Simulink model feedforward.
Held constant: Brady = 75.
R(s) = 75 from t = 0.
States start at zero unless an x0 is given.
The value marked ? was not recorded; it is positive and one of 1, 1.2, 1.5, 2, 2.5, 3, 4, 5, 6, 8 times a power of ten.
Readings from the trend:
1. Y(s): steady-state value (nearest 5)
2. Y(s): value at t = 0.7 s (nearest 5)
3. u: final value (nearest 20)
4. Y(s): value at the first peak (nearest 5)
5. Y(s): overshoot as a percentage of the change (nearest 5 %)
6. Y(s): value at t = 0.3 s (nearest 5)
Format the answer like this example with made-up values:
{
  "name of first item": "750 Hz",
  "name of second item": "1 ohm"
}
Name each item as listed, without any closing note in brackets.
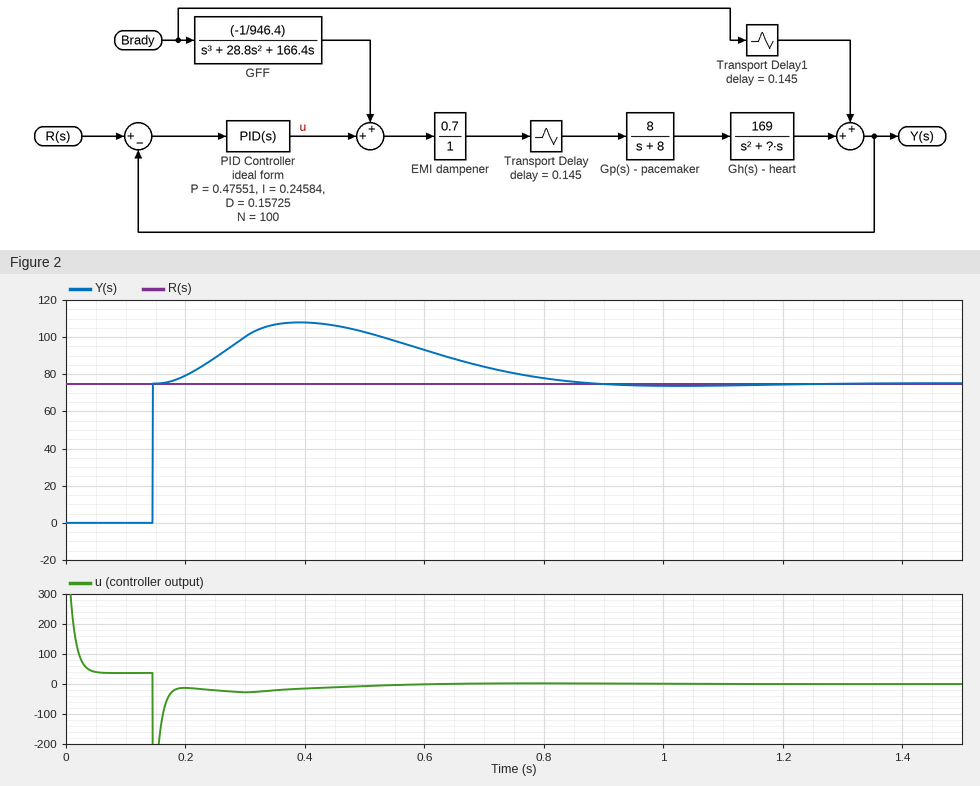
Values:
{
  "Y(s): steady-state value": "75",
  "Y(s): value at t = 0.7 s": "85",
  "u: final value": "0",
  "Y(s): value at the first peak": "110",
  "Y(s): overshoot as a percentage of the change": "45 %",
  "Y(s): value at t = 0.3 s": "100"
}
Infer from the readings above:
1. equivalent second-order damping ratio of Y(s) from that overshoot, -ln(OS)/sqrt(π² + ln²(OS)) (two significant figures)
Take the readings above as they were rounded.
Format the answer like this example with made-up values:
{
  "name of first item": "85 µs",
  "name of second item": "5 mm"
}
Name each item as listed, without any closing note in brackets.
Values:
{
  "equivalent second-order damping ratio of Y(s) from that overshoot, -ln(OS)/sqrt(π² + ln²(OS))": "0.25"
}
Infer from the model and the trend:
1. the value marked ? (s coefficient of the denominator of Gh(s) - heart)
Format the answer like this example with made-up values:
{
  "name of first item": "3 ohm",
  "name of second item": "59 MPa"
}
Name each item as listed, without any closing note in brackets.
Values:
{
  "the value marked ? (s coefficient of the denominator of Gh(s) - heart)": "20"
}
